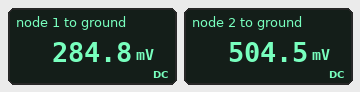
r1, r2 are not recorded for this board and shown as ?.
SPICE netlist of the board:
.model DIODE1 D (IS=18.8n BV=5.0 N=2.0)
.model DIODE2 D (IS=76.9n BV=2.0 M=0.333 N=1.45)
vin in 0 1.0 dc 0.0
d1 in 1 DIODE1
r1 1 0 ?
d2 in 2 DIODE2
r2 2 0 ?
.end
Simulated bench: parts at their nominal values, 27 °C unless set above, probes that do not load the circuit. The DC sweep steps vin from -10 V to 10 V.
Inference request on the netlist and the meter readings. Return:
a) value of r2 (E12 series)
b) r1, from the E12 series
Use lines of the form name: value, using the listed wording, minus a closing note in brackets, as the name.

value of r2: 12 Ω
r1, from the E12 series: 15 Ω
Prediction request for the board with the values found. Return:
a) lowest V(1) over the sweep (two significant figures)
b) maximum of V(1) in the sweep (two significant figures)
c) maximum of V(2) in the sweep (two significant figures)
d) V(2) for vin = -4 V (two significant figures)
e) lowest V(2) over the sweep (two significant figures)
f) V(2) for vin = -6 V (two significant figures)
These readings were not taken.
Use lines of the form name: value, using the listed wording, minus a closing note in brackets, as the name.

lowest V(1) over the sweep: -4.7 V
maximum of V(1) in the sweep: 9.1 V
maximum of V(2) in the sweep: 9.4 V
V(2) for vin = -4 V: -1.8 V
lowest V(2) over the sweep: -7.8 V
V(2) for vin = -6 V: -3.8 V
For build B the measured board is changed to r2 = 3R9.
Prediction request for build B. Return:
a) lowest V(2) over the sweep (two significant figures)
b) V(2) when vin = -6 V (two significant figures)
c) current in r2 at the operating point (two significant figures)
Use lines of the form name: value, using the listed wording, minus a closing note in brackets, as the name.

lowest V(2) over the sweep: -7.7 V
V(2) when vin = -6 V: -3.7 V
current in r2 at the operating point: 120 mA
